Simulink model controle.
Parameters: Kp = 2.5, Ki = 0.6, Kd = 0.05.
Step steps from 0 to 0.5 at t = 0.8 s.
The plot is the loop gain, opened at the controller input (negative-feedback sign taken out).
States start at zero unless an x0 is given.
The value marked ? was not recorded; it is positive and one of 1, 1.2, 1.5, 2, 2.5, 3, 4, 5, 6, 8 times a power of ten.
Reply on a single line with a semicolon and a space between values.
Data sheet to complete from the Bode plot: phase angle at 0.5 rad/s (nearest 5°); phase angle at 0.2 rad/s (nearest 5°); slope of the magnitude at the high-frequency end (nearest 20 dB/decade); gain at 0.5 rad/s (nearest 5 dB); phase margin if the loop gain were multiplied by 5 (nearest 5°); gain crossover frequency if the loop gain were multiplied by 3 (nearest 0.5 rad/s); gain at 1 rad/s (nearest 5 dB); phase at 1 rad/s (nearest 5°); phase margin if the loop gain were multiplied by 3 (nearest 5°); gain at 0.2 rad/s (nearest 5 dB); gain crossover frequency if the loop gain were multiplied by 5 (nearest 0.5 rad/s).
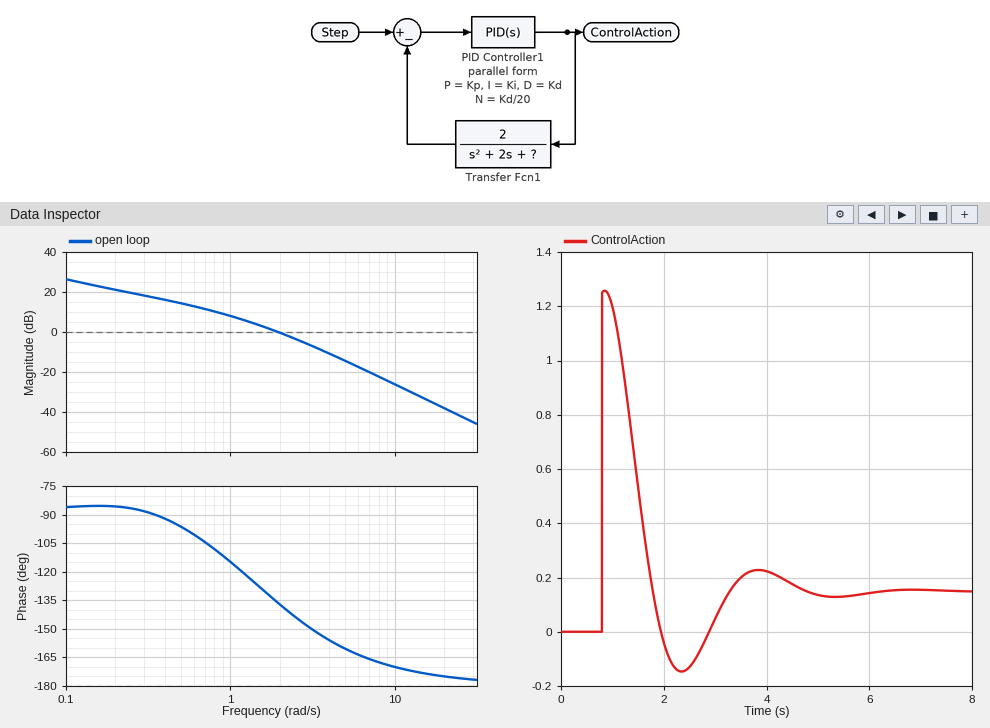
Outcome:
-95°; -85°; -40 dB/decade; 15 dB; 20°; 3.5 rad/s; 10 dB; -115°; 25°; 20 dB; 5.0 rad/s
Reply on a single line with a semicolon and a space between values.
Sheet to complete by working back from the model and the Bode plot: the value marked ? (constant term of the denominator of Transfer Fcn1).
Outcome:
0.6
